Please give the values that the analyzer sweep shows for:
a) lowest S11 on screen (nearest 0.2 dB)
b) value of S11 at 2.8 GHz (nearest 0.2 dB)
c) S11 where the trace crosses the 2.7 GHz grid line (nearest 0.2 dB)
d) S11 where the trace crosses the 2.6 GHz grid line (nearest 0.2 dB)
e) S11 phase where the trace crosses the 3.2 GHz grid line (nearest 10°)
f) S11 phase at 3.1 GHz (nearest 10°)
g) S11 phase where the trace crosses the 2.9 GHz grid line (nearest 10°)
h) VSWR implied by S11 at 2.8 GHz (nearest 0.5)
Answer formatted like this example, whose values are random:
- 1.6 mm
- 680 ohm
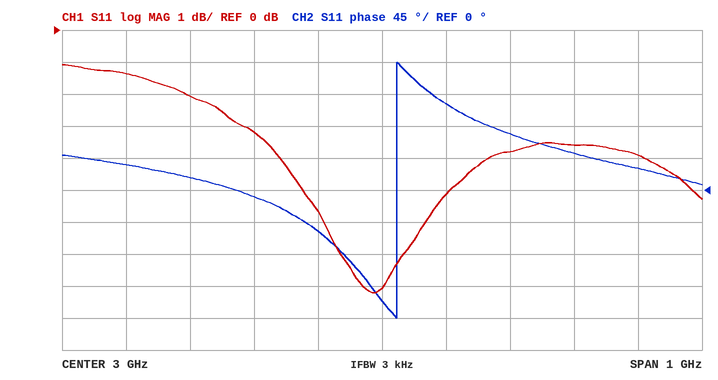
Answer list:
- -8.2 dB
- -3.2 dB
- -2.0 dB
- -1.4 dB
- 80°
- 120°
- -60°
- 5.5
